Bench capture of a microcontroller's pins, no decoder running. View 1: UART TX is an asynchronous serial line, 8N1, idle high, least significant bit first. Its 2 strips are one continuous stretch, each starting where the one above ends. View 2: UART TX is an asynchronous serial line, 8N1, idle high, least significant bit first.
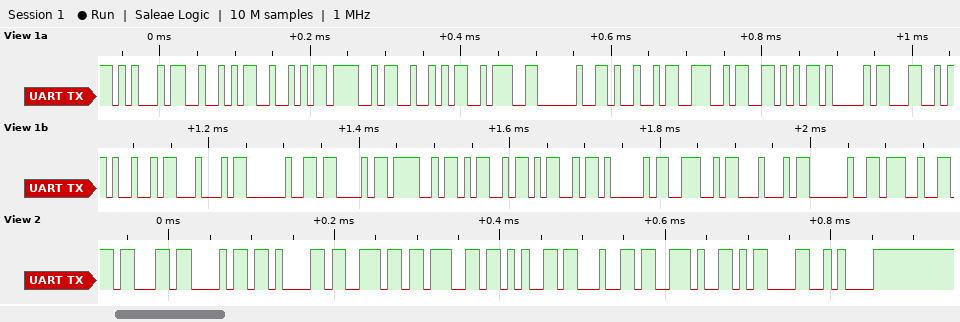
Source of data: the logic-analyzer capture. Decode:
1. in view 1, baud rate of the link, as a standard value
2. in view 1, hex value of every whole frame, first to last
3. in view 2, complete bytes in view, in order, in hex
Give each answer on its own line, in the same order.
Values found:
115200 baud
45 52 52 4F 52 3A 20 49 4E 56 41 4C 49 44 20 43 4F 4D 4D 41 4E 44 20 27
63 68 61 6E 67 65 64 2E 0D 0A
